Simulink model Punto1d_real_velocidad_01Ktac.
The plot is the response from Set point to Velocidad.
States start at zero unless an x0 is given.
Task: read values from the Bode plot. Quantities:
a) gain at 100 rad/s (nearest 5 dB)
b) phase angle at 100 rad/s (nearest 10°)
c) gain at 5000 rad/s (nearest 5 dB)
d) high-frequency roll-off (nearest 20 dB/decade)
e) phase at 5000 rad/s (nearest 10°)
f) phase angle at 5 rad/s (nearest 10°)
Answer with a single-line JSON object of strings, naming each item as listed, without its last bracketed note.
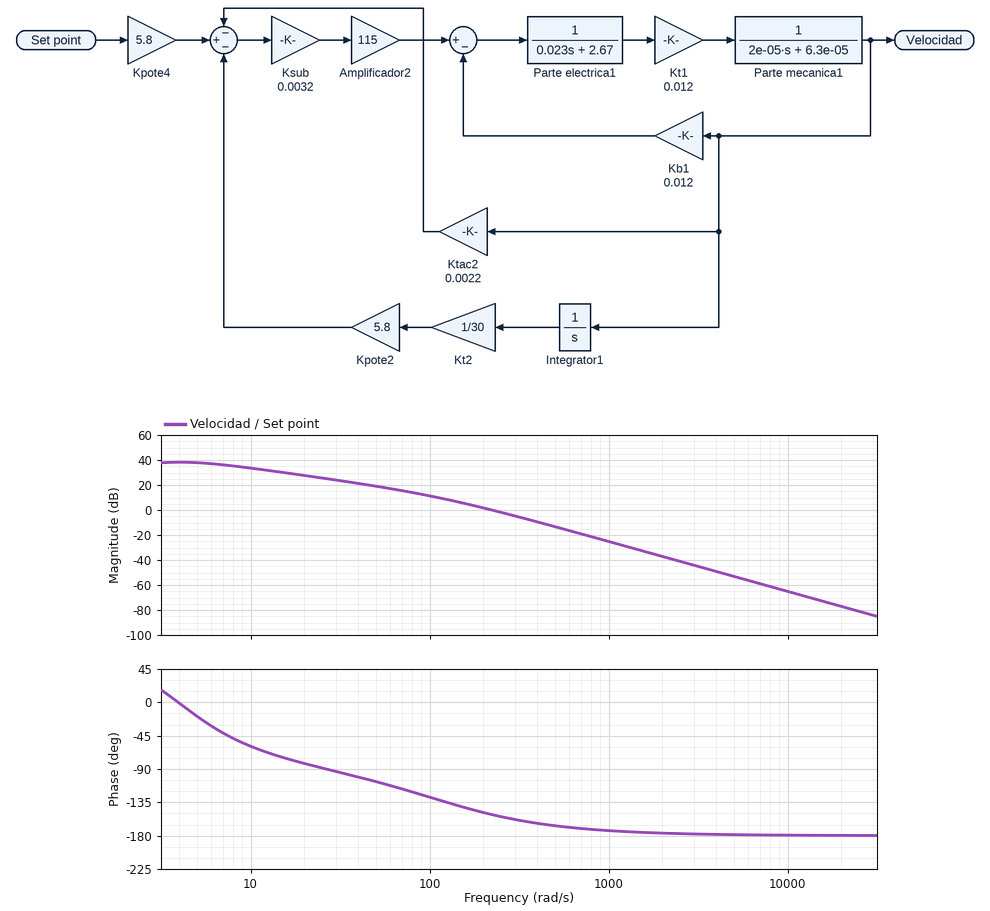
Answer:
{"gain at 100 rad/s": "10 dB", "phase angle at 100 rad/s": "-130°", "gain at 5000 rad/s": "-55 dB", "high-frequency roll-off": "-40 dB/decade", "phase at 5000 rad/s": "-180°", "phase angle at 5 rad/s": "-20°"}
